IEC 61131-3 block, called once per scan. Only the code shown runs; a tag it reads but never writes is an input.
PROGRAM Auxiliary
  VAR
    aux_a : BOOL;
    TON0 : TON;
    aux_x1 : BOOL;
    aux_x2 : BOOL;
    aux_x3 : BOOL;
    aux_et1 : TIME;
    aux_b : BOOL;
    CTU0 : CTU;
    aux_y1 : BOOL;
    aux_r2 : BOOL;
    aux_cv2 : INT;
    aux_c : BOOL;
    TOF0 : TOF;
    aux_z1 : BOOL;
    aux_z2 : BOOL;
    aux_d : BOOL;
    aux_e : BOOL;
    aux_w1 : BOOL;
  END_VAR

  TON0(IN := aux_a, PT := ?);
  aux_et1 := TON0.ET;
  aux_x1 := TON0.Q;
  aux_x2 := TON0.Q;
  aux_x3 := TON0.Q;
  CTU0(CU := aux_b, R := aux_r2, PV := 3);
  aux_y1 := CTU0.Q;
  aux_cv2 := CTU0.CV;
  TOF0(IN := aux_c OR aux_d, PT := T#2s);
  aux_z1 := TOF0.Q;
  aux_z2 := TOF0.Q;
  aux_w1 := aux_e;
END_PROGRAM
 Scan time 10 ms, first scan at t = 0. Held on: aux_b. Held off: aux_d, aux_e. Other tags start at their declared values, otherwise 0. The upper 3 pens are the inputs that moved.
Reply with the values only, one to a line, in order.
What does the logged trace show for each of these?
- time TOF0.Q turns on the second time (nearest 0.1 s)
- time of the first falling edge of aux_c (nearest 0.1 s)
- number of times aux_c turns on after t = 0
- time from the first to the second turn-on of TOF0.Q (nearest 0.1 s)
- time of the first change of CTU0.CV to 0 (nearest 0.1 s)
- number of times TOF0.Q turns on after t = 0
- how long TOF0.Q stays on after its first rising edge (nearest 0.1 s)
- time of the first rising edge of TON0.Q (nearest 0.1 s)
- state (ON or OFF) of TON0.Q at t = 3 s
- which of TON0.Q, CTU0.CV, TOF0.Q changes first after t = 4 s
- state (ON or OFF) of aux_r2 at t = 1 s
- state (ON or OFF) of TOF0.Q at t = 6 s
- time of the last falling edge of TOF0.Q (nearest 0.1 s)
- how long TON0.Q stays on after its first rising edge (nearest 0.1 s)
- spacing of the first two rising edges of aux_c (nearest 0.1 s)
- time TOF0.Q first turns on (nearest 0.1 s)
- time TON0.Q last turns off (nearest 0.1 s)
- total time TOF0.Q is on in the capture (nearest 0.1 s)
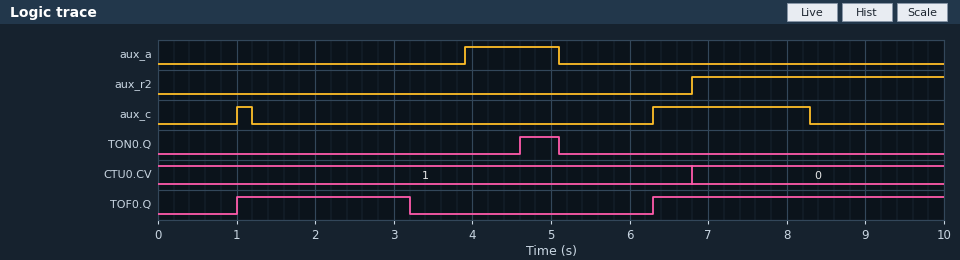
6.3 s
1.2 s
2
5.3 s
6.8 s
2
2.2 s
4.6 s
OFF
TON0.Q
OFF
OFF
3.2 s
0.5 s
5.3 s
1.0 s
5.1 s
5.9 s
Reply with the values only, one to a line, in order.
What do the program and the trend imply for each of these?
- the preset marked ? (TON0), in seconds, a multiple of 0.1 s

0.7 s
